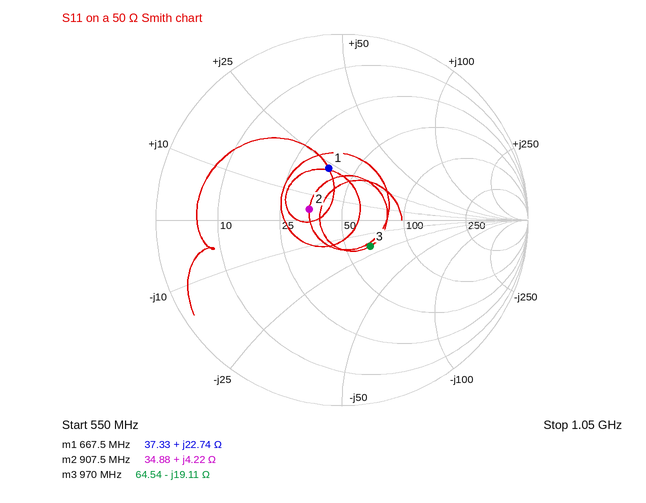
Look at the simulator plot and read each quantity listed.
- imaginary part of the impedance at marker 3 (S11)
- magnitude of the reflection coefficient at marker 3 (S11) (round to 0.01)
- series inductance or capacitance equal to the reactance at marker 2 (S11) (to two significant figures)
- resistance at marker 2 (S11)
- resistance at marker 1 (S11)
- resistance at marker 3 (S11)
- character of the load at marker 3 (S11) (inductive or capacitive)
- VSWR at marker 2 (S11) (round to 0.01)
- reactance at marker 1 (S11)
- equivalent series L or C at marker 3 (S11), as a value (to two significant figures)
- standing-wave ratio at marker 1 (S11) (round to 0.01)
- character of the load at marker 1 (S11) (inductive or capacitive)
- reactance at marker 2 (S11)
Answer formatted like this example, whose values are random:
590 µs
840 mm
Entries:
-19.11 Ω
0.21
740 pH
34.88 Ω
37.33 Ω
64.54 Ω
capacitive
1.45
+22.74 Ω
8.6 pF
1.81
inductive
+4.22 Ω
